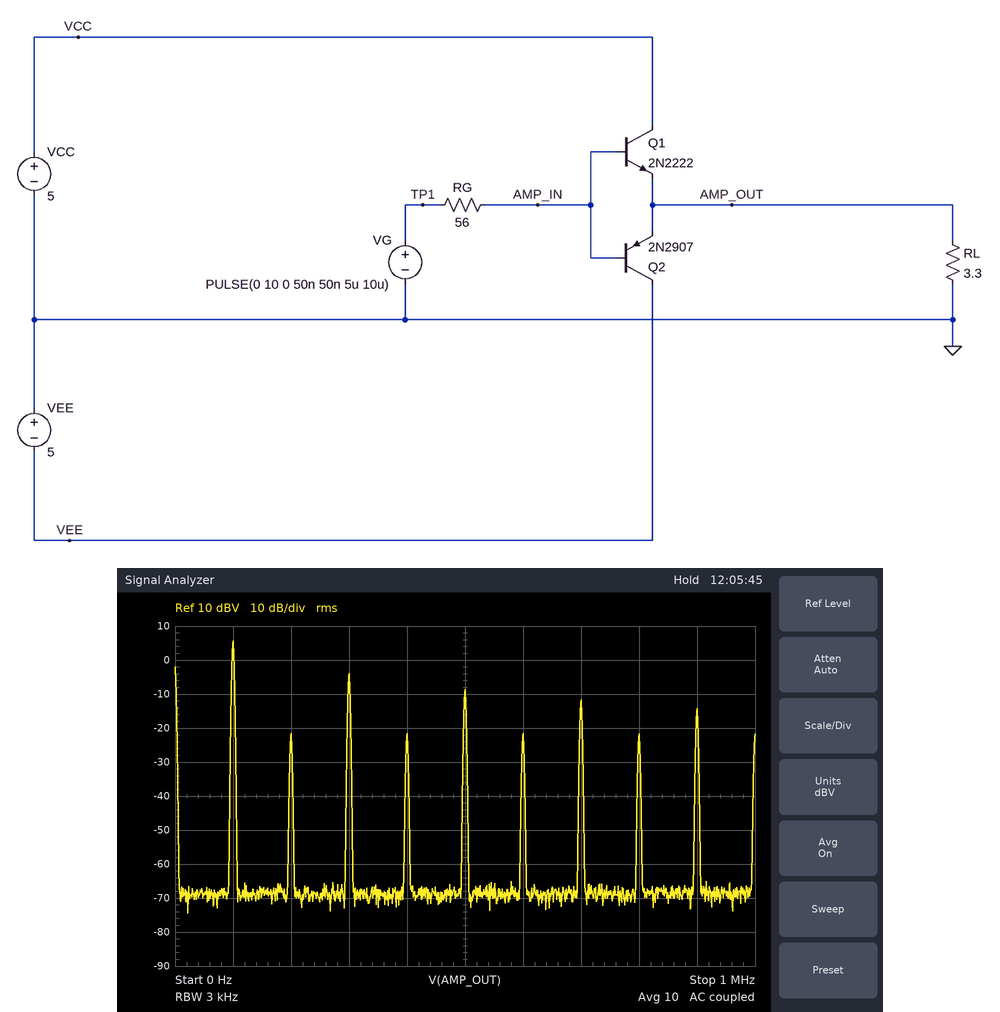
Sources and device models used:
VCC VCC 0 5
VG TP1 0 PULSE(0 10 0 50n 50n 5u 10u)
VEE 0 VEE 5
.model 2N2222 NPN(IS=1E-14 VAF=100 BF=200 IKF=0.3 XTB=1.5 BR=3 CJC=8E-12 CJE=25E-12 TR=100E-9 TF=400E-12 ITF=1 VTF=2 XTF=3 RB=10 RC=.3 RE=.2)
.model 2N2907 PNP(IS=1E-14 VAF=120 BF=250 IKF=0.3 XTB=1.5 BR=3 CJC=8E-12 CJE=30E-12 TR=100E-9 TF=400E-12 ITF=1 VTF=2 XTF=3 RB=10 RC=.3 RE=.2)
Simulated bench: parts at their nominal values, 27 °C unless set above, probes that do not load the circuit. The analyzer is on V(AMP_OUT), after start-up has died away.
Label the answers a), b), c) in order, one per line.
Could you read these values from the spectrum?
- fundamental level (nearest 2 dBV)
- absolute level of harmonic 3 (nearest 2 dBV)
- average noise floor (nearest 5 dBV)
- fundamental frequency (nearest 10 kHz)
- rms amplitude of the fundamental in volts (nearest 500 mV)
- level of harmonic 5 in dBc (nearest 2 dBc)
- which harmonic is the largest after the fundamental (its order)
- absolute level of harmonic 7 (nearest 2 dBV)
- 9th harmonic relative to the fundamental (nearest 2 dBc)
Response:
a) 6 dBV
b) -4 dBV
c) -70 dBV
d) 100 kHz
e) 2.0 V
f) -14 dBc
g) 3
h) -12 dBV
i) -20 dBc
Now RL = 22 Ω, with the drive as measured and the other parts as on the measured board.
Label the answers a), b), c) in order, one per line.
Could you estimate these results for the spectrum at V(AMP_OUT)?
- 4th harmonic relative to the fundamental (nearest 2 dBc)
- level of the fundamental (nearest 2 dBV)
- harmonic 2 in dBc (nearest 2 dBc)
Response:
a) -24 dBc
b) 6 dBV
c) -24 dBc
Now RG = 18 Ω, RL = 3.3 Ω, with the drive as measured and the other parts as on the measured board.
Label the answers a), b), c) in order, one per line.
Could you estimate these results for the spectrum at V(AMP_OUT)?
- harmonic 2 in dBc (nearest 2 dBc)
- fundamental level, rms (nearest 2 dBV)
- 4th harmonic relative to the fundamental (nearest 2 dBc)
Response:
a) -24 dBc
b) 6 dBV
c) -24 dBc
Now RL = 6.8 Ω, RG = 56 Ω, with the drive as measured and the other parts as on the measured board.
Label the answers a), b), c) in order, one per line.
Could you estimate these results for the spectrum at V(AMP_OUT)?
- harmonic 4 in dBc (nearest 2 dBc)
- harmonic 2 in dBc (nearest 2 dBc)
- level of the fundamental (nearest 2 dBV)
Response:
a) -24 dBc
b) -24 dBc
c) 6 dBV
